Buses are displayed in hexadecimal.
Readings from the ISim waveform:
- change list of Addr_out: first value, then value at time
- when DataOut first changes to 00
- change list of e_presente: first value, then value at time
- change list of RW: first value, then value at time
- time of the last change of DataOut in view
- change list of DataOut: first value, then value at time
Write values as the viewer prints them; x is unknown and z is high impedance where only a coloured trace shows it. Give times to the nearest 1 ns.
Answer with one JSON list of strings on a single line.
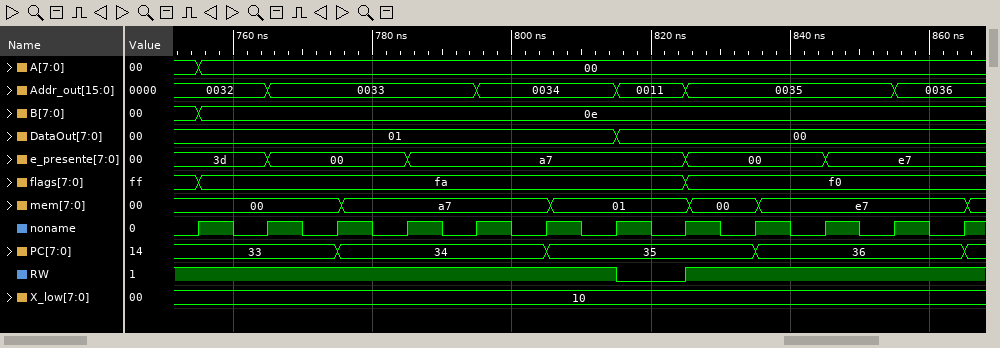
["0032, 0033 at 765 ns, 0034 at 795 ns, 0011 at 815 ns, 0035 at 825 ns, 0036 at 855 ns", "815 ns", "3d, 00 at 765 ns, a7 at 785 ns, 00 at 825 ns, e7 at 845 ns", "1, 0 at 815 ns, 1 at 825 ns", "815 ns", "01, 00 at 815 ns"]
